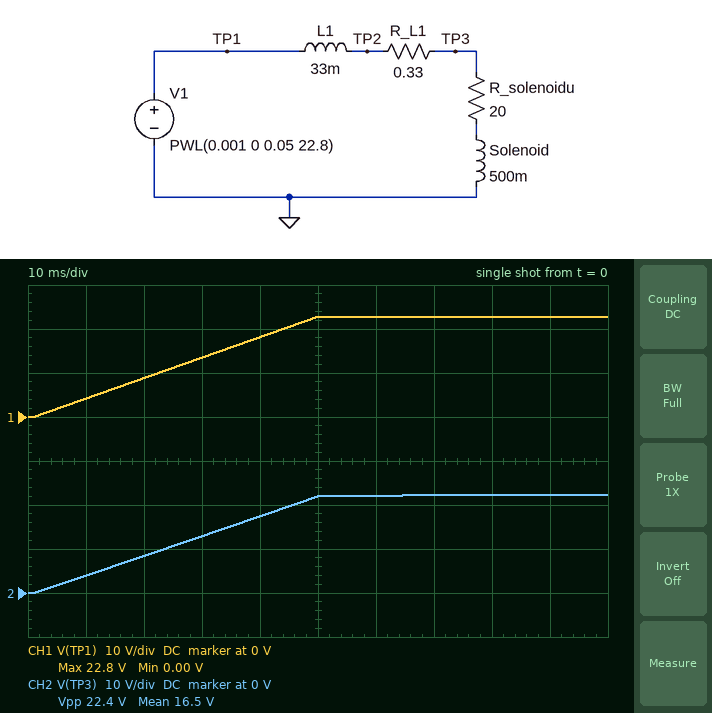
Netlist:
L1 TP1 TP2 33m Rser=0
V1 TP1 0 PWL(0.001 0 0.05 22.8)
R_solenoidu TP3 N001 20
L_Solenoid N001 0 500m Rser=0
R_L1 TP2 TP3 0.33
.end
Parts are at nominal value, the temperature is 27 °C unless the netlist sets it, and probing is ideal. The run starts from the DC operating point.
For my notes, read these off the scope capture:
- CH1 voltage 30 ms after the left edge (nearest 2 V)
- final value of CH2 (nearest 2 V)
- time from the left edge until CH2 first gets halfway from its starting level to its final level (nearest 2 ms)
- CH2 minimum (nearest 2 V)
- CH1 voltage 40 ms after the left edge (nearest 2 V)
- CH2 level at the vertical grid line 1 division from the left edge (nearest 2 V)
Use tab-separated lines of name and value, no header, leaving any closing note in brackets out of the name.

CH1 voltage 30 ms after the left edge	14 V
final value of CH2	22 V
time from the left edge until CH2 first gets halfway from its starting level to its final level	26 ms
CH2 minimum	0 V
CH1 voltage 40 ms after the left edge	18 V
CH2 level at the vertical grid line 1 division from the left edge	4 V
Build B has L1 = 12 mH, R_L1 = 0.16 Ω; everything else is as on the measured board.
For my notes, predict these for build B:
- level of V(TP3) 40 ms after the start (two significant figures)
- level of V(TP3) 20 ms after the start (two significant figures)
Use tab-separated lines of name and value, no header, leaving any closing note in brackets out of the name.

level of V(TP3) 40 ms after the start	18 V
level of V(TP3) 20 ms after the start	8.7 V
